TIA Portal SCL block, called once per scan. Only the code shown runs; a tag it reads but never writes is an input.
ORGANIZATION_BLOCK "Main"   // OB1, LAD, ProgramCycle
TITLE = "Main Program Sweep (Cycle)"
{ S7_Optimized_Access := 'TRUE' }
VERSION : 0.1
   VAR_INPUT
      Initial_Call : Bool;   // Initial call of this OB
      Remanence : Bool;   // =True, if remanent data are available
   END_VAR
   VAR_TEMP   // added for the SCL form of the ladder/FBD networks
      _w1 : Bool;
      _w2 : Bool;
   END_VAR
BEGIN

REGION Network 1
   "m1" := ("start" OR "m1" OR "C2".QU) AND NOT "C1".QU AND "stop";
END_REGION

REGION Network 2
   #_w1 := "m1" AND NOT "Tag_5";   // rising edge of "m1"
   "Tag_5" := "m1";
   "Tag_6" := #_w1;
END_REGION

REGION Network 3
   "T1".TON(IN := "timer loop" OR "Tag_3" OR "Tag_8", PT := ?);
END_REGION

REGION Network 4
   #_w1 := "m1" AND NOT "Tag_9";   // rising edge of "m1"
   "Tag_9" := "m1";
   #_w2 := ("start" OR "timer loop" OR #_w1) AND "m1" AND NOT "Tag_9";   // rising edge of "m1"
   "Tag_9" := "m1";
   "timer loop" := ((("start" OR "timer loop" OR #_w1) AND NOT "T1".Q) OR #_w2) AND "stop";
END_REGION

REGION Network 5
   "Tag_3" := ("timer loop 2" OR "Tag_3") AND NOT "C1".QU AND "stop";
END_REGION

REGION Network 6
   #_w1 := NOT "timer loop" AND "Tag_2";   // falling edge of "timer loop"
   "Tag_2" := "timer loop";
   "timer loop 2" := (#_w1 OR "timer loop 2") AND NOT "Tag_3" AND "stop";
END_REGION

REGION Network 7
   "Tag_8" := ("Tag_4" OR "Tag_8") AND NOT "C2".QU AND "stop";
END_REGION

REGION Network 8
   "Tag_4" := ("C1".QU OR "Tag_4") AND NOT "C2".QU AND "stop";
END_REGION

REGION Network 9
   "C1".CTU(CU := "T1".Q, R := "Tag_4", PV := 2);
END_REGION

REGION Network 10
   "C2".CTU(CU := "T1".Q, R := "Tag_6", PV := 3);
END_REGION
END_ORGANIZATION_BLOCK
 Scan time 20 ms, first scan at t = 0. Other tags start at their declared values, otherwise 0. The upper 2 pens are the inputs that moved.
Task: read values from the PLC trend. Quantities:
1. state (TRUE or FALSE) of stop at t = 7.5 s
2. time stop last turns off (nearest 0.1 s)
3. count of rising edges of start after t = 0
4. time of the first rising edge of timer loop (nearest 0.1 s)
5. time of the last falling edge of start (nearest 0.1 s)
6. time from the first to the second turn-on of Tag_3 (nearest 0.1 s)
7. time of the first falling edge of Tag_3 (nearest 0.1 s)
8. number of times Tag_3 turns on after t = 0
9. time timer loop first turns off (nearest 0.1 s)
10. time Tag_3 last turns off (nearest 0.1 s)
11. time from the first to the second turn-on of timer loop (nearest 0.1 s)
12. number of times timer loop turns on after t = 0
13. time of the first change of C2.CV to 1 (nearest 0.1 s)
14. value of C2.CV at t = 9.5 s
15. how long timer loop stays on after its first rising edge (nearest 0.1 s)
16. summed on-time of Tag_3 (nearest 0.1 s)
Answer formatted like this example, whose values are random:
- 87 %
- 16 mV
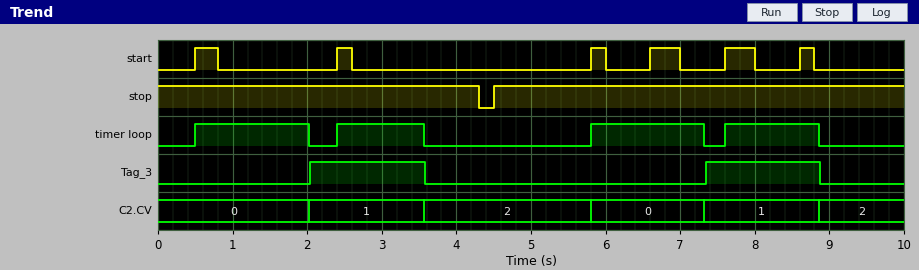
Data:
- TRUE
- 4.3 s
- 6
- 0.5 s
- 8.8 s
- 5.3 s
- 3.6 s
- 2
- 2.0 s
- 8.9 s
- 1.9 s
- 4
- 2.0 s
- 2
- 1.5 s
- 3.1 s
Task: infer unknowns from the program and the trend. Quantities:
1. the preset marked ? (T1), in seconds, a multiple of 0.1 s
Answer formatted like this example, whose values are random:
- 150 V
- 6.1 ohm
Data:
- 1.5 s
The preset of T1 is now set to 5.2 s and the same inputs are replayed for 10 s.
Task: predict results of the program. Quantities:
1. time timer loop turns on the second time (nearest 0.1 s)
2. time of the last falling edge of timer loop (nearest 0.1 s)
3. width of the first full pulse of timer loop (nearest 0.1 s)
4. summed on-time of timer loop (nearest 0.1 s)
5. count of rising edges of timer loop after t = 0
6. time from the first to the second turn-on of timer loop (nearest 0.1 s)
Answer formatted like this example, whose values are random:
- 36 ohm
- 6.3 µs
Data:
- 5.8 s
- 4.3 s
- 3.8 s
- 8.0 s
- 2
- 5.3 s
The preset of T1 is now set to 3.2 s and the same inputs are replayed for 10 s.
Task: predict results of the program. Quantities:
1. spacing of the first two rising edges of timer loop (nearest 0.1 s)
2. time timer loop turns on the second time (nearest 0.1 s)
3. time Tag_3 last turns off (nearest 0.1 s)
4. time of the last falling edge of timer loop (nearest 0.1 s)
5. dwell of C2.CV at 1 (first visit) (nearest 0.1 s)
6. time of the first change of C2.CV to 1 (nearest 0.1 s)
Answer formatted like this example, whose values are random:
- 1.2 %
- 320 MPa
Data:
- 5.3 s
- 5.8 s
- 4.3 s
- 9.0 s
- 2.1 s
- 3.7 s
